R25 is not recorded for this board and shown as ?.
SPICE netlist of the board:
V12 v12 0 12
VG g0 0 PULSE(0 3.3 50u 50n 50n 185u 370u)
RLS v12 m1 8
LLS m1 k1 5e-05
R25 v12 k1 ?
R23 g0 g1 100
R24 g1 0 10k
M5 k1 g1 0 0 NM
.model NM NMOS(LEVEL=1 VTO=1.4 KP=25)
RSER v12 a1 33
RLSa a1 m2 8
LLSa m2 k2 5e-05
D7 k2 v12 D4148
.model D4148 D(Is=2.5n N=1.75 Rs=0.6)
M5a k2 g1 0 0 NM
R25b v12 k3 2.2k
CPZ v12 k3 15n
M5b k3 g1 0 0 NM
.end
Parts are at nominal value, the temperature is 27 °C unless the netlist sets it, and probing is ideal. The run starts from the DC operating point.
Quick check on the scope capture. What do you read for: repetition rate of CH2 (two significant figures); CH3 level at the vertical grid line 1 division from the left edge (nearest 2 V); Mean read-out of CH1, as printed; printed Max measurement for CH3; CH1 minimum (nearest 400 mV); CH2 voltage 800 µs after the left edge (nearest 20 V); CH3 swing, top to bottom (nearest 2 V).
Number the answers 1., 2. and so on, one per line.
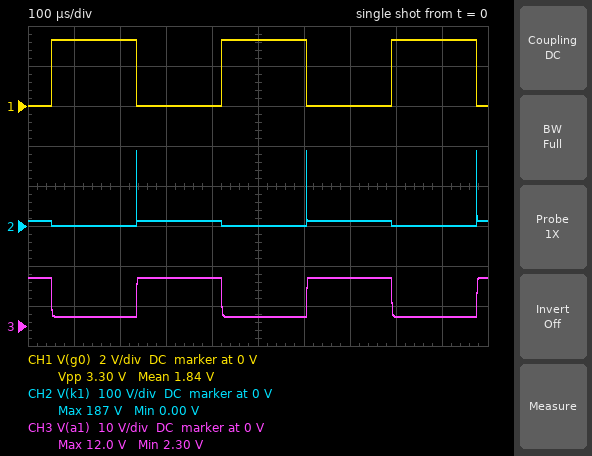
1. 2.7 kHz
2. 2 V
3. 1.84 V
4. 12.0 V
5. 0 V
6. 0 V
7. 10 V
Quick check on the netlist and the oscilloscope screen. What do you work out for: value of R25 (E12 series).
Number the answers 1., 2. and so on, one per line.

1. 120 Ω
